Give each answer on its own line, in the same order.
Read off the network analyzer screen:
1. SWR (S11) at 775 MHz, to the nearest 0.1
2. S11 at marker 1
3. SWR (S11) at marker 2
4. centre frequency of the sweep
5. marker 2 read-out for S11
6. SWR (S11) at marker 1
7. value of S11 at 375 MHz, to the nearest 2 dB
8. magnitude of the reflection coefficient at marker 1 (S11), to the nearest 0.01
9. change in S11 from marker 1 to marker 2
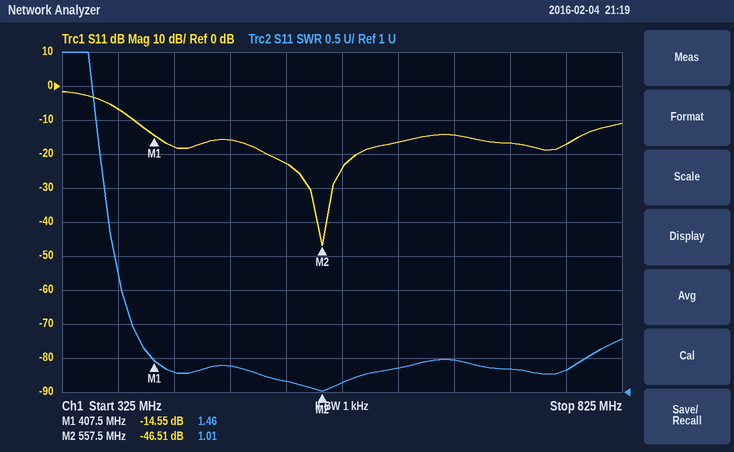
1.3
-14.55 dB
1.01
575 MHz
-46.51 dB
1.46
-6 dB
0.19
-31.96 dB
